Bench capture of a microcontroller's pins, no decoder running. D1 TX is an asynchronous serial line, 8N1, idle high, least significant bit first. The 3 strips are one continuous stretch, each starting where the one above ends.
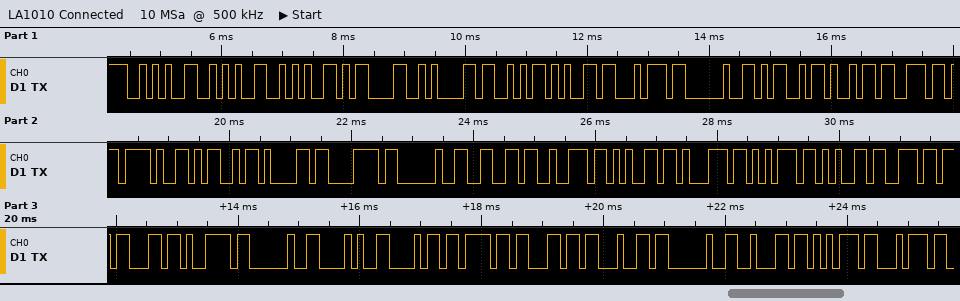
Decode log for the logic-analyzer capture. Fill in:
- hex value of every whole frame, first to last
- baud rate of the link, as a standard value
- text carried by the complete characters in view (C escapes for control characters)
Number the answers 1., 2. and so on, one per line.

1. 0x2A 0x2A 0x2A 0x0D 0x0A 0x53 0x65 0x74 0x20 0x4D 0x69 0x6E 0x2F 0x4D 0x61 0x78 0x20 0x66 0x72 0x65 0x71 0x75 0x65 0x6E 0x63 0x79 0x20 0x28 0x68 0x6F 0x6C 0x64 0x20 0x62 0x75 0x74
2. 9600 baud
3. "***\r\nSet Min/Max frequency (hold but"
